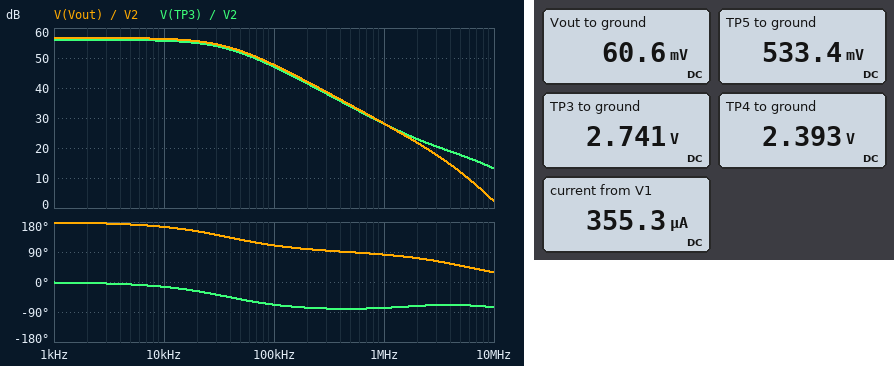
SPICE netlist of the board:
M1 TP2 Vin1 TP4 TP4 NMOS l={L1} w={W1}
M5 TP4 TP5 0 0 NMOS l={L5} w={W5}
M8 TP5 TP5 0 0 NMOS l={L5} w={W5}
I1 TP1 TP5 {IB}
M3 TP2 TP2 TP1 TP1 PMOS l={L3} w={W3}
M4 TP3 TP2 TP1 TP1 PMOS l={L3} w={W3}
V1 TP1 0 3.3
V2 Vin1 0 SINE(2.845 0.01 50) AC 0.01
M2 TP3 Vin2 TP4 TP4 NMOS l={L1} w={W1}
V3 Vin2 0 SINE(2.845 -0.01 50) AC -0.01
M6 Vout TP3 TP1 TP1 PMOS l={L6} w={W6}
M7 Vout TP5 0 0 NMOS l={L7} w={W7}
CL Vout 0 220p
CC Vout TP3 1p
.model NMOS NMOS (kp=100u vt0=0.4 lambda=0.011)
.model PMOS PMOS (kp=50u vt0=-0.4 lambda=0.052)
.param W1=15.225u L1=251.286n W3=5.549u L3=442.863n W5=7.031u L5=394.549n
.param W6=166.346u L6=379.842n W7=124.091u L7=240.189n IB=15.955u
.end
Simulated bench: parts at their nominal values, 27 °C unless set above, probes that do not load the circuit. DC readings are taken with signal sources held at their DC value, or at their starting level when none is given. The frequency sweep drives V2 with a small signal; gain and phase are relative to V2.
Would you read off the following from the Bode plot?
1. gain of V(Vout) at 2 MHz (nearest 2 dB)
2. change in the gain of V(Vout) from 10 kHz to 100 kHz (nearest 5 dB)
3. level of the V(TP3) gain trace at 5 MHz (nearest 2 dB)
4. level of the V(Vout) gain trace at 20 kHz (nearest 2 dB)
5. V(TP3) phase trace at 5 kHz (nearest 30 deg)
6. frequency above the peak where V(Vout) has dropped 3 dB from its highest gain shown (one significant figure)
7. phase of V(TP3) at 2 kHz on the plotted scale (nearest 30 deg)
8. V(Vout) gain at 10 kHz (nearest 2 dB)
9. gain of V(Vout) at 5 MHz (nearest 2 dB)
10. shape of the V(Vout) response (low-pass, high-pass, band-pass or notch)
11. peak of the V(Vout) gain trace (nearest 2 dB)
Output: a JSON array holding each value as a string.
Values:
["22 dB", "-10 dB", "18 dB", "56 dB", "0 deg", "40 kHz", "0 deg", "56 dB", "12 dB", "low-pass", "56 dB"]
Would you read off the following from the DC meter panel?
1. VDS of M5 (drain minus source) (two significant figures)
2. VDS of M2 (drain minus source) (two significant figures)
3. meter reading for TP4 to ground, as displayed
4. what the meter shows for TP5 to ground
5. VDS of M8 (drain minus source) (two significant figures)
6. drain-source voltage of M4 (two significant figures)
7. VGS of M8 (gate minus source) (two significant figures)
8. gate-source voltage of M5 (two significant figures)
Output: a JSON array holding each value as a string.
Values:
["2.4 V", "350 mV", "2.393 V", "533.4 mV", "530 mV", "-560 mV", "530 mV", "530 mV"]
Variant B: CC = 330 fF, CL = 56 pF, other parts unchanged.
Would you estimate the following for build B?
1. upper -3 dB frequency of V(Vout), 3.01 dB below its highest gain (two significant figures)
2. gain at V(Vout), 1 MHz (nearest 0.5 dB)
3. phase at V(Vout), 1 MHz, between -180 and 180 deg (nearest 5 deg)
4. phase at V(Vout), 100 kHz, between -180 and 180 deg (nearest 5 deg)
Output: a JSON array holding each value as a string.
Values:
["120 kHz", "38.0 dB", "95 deg", "140 deg"]
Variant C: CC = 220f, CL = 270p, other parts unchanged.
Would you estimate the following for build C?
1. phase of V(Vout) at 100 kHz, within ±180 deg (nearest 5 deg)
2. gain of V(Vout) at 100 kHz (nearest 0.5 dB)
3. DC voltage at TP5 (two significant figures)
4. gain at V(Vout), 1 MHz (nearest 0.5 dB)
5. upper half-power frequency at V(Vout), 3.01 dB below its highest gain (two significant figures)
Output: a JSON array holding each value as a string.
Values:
["150 deg", "55.5 dB", "530 mV", "41.0 dB", "170 kHz"]
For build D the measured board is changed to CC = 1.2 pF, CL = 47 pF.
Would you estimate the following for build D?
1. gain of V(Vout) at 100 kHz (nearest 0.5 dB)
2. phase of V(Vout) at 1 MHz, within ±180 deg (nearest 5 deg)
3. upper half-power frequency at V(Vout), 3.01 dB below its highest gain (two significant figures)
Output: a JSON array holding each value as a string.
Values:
["46.5 dB", "90 deg", "32 kHz"]
